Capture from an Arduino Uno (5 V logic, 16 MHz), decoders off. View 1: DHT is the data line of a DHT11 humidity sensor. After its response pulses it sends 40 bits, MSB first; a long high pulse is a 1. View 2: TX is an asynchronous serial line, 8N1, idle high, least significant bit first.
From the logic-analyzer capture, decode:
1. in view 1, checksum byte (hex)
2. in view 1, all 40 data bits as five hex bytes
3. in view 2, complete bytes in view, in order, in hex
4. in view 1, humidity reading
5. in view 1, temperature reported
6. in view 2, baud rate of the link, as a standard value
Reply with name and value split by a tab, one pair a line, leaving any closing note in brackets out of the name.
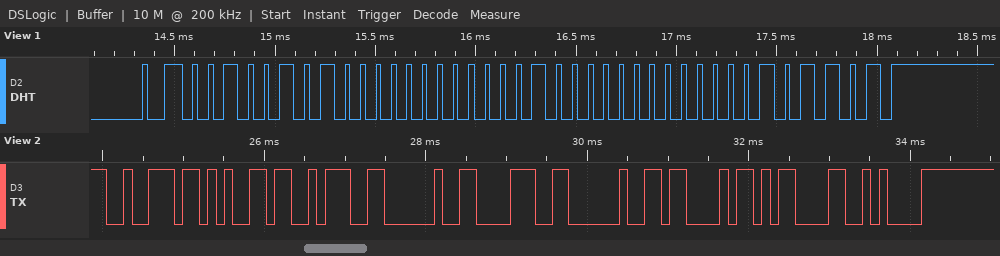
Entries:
in view 1, checksum byte	0x2D
in view 1, all 40 data bits as five hex bytes	25 00 08 00 2D
in view 2, complete bytes in view, in order, in hex	72 65 3A 20 38 20 43 0D 0A
in view 1, humidity reading	37 %
in view 1, temperature reported	8.0 °C
in view 2, baud rate of the link, as a standard value	9600 baud
